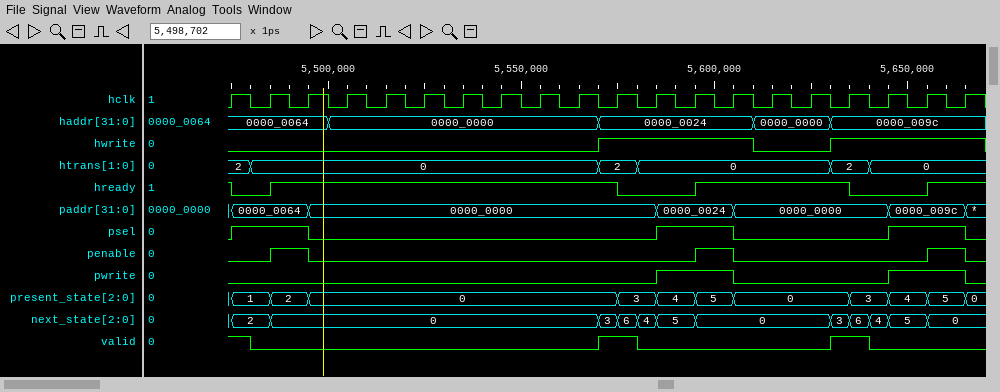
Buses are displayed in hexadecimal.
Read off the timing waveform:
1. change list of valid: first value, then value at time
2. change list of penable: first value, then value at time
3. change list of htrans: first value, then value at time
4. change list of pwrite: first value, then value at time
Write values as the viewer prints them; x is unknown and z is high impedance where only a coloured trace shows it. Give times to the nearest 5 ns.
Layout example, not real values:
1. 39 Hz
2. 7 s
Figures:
1. 1, 0 at 5480 ns, 1 at 5570 ns, 0 at 5580 ns, 1 at 5630 ns, 0 at 5640 ns
2. 0, 1 at 5485 ns, 0 at 5495 ns, 1 at 5595 ns, 0 at 5605 ns, 1 at 5655 ns, 0 at 5665 ns
3. 2, 0 at 5480 ns, 2 at 5570 ns, 0 at 5580 ns, 2 at 5630 ns, 0 at 5640 ns
4. 0, 1 at 5585 ns, 0 at 5605 ns, 1 at 5645 ns, 0 at 5665 ns
